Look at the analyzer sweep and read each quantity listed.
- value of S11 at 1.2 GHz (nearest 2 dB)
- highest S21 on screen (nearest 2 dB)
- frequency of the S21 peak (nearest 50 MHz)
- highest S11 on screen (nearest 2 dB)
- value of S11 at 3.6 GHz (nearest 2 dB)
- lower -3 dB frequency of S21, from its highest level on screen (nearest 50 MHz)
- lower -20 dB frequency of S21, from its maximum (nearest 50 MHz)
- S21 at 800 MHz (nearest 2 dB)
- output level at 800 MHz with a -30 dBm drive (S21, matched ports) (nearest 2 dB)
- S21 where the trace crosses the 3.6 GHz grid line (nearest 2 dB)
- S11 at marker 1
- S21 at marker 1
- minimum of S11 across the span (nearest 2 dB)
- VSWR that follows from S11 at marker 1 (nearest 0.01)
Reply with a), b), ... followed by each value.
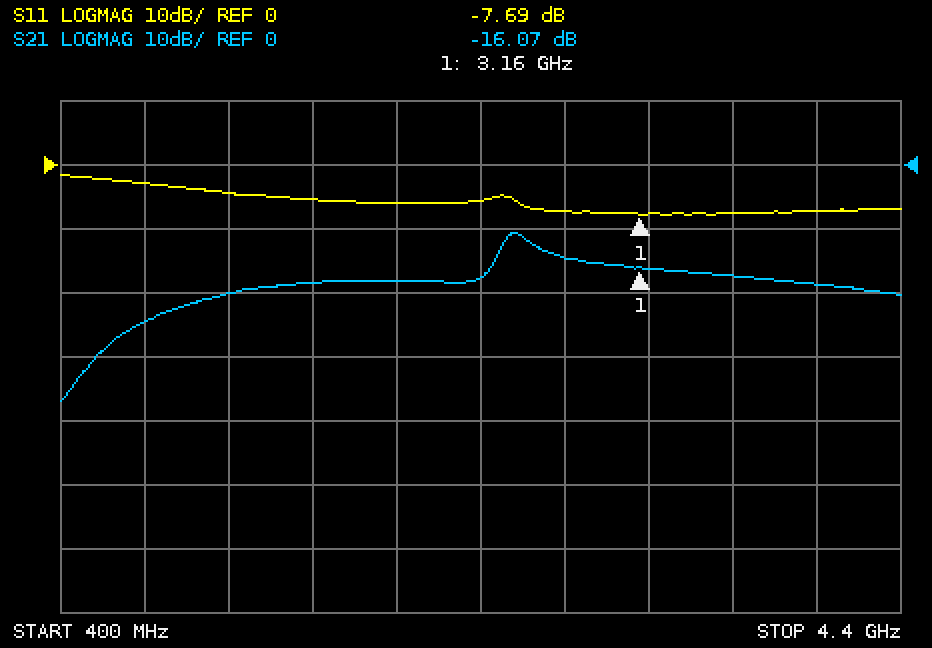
a) -4 dB
b) -10 dB
c) 2.55 GHz
d) -2 dB
e) -8 dB
f) 2.50 GHz
g) 550 MHz
h) -24 dB
i) -54 dBm
j) -18 dB
k) -7.69 dB
l) -16.07 dB
m) -8 dB
n) 2.40
